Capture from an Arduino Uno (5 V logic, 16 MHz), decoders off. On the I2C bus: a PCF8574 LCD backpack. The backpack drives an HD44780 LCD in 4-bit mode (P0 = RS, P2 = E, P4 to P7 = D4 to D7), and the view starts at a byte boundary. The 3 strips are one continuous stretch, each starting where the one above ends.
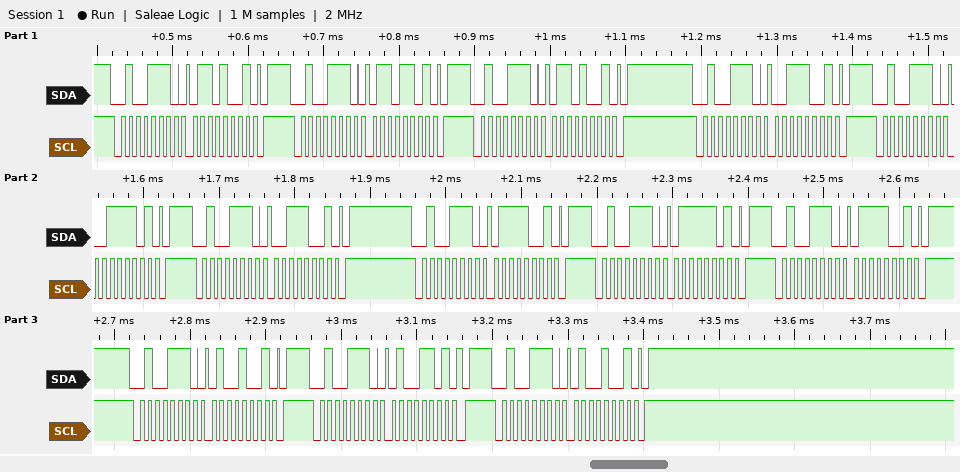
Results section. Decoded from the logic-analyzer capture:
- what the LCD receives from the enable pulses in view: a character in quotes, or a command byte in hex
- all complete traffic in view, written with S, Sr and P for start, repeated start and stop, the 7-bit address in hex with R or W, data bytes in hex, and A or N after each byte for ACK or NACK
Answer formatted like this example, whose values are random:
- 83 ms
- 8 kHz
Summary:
- 'c' 't'
- S 27W A 69 A P S 27W A 6D A P S 27W A 69 A P S 27W A 39 A P S 27W A 3D A P S 27W A 39 A P S 27W A 79 A P S 27W A 7D A P S 27W A 79 A P S 27W A 49 A P S 27W A 4D A P S 27W A 49 A P
